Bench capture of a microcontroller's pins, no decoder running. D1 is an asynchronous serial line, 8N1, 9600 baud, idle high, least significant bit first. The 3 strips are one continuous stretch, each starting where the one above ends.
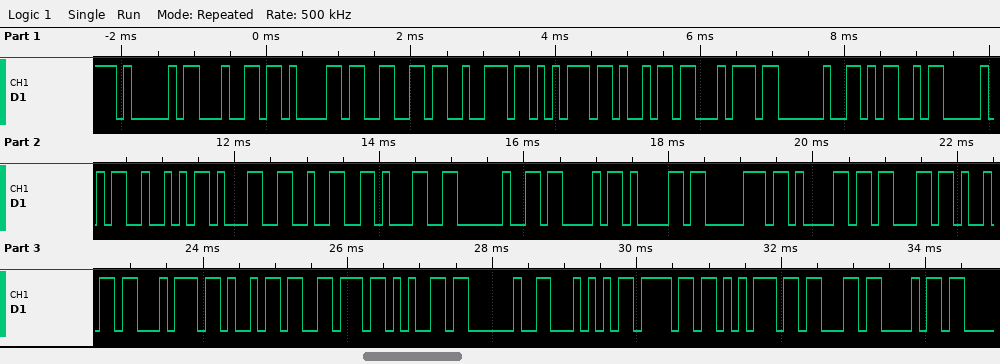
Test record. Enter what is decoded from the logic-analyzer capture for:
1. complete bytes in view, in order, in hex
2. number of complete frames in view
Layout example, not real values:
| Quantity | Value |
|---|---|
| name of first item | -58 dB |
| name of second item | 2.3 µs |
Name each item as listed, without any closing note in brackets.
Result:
| Quantity | Value |
|---|---|
| complete bytes in view, in order, in hex | 41 64 61 66 72 75 69 74 20 4D 50 52 31 32 31 20 43 61 70 61 63 69 74 69 76 65 20 54 6F 75 63 68 |
| number of complete frames in view | 32 |
